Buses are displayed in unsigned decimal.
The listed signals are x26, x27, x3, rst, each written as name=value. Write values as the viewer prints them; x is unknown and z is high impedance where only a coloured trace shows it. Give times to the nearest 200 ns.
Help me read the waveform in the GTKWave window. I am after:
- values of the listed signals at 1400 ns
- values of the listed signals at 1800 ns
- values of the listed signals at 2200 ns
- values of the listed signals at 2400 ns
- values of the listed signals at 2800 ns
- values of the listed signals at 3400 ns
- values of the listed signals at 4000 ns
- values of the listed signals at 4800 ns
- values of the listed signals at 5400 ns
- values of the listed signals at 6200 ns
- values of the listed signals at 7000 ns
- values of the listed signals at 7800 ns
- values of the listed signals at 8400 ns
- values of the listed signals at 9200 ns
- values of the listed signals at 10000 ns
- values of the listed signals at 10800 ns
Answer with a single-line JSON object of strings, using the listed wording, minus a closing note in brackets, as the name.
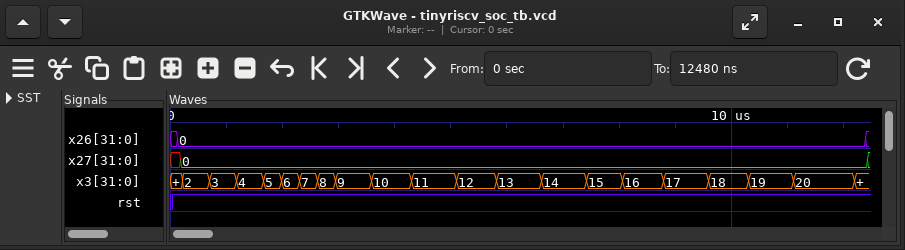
{"values of the listed signals at 1400 ns": "x26=0, x27=0, x3=4, rst=1", "values of the listed signals at 1800 ns": "x26=0, x27=0, x3=5, rst=1", "values of the listed signals at 2200 ns": "x26=0, x27=0, x3=6, rst=1", "values of the listed signals at 2400 ns": "x26=0, x27=0, x3=7, rst=1", "values of the listed signals at 2800 ns": "x26=0, x27=0, x3=8, rst=1", "values of the listed signals at 3400 ns": "x26=0, x27=0, x3=9, rst=1", "values of the listed signals at 4000 ns": "x26=0, x27=0, x3=10, rst=1", "values of the listed signals at 4800 ns": "x26=0, x27=0, x3=11, rst=1", "values of the listed signals at 5400 ns": "x26=0, x27=0, x3=12, rst=1", "values of the listed signals at 6200 ns": "x26=0, x27=0, x3=13, rst=1", "values of the listed signals at 7000 ns": "x26=0, x27=0, x3=14, rst=1", "values of the listed signals at 7800 ns": "x26=0, x27=0, x3=15, rst=1", "values of the listed signals at 8400 ns": "x26=0, x27=0, x3=16, rst=1", "values of the listed signals at 9200 ns": "x26=0, x27=0, x3=17, rst=1", "values of the listed signals at 10000 ns": "x26=0, x27=0, x3=18, rst=1", "values of the listed signals at 10800 ns": "x26=0, x27=0, x3=19, rst=1"}
